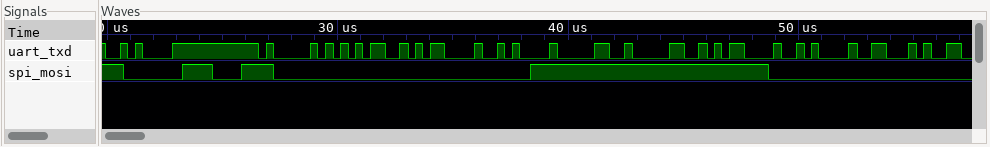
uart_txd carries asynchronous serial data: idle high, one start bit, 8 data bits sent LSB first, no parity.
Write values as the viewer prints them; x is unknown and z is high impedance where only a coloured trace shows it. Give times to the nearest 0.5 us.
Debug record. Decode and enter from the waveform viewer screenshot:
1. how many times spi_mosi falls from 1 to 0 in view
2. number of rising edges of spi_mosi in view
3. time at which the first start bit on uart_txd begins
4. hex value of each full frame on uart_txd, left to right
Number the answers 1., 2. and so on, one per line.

1. 4
2. 3
3. 20 us
4. 0A, 41, 35, 0D, 0A, 30, 30, 0D, 0A, 46
